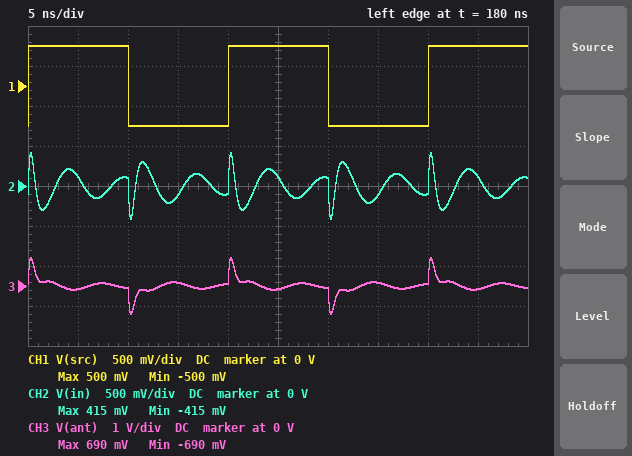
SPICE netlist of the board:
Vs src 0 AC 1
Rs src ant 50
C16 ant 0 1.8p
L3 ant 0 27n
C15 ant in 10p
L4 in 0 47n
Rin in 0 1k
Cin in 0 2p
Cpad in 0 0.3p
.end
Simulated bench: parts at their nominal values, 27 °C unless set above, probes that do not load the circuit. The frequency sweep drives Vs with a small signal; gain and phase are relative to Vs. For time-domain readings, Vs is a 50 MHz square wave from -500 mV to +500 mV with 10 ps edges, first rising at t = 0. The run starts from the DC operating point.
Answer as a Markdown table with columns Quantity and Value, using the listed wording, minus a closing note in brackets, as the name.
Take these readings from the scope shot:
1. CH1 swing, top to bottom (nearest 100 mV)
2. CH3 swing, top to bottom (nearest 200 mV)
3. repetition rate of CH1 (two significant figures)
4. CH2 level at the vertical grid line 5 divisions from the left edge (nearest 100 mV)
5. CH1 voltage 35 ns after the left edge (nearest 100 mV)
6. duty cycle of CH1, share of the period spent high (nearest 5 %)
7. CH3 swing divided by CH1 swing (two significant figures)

| Quantity | Value |
|---|---|
| CH1 swing, top to bottom | 1.0 V |
| CH3 swing, top to bottom | 1.4 V |
| repetition rate of CH1 | 50 MHz |
| CH2 level at the vertical grid line 5 divisions from the left edge | 100 mV |
| CH1 voltage 35 ns after the left edge | -500 mV |
| duty cycle of CH1, share of the period spent high | 50 % |
| CH3 swing divided by CH1 swing | 1.4 |
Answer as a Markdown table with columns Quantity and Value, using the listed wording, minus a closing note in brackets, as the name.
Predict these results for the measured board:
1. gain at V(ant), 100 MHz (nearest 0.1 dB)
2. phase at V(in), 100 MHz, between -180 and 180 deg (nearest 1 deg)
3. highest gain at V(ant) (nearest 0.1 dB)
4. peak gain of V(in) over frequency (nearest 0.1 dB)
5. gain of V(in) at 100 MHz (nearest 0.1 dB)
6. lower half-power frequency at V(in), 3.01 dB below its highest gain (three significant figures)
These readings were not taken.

| Quantity | Value |
|---|---|
| gain at V(ant), 100 MHz | -8.6 dB |
| phase at V(in), 100 MHz, between -180 and 180 deg | -114 deg |
| highest gain at V(ant) | -0.4 dB |
| peak gain of V(in) over frequency | 5.2 dB |
| gain of V(in) at 100 MHz | -21.0 dB |
| lower half-power frequency at V(in), 3.01 dB below its highest gain | 169 MHz |
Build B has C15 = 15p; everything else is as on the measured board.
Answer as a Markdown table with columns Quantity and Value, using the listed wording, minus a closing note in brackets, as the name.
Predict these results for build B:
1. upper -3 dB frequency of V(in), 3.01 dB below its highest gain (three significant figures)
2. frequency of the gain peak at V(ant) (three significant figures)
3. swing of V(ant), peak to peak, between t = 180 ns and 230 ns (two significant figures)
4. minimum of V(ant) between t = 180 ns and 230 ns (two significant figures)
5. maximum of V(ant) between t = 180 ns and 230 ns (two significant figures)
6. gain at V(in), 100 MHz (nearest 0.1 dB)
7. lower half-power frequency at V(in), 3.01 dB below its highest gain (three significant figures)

| Quantity | Value |
|---|---|
| upper -3 dB frequency of V(in), 3.01 dB below its highest gain | 172 MHz |
| frequency of the gain peak at V(ant) | 608 MHz |
| swing of V(ant), peak to peak, between t = 180 ns and 230 ns | 1.1 V |
| minimum of V(ant) between t = 180 ns and 230 ns | -570 mV |
| maximum of V(ant) between t = 180 ns and 230 ns | 570 mV |
| gain at V(in), 100 MHz | -15.5 dB |
| lower half-power frequency at V(in), 3.01 dB below its highest gain | 140 MHz |
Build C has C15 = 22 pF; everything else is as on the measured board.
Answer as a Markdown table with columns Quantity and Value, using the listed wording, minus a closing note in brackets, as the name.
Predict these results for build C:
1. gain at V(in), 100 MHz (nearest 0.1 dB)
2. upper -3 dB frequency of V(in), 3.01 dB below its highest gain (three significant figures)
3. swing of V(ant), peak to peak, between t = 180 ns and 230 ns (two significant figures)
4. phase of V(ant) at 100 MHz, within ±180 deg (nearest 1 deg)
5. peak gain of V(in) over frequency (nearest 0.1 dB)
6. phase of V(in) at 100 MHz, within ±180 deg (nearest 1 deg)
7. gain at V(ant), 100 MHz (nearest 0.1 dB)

| Quantity | Value |
|---|---|
| gain at V(in), 100 MHz | -8.5 dB |
| upper -3 dB frequency of V(in), 3.01 dB below its highest gain | 139 MHz |
| swing of V(ant), peak to peak, between t = 180 ns and 230 ns | 1.2 V |
| phase of V(ant) at 100 MHz, within ±180 deg | 59 deg |
| peak gain of V(in) over frequency | 4.4 dB |
| phase of V(in) at 100 MHz, within ±180 deg | -124 deg |
| gain at V(ant), 100 MHz | -5.9 dB |
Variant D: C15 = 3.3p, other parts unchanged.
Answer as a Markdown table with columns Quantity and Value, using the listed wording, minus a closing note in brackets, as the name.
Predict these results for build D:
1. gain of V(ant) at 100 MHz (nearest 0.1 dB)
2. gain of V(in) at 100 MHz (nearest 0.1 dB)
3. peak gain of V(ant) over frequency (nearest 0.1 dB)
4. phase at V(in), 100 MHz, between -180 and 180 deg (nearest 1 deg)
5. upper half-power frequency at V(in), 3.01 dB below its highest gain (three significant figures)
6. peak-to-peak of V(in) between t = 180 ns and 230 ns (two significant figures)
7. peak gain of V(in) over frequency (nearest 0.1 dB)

| Quantity | Value |
|---|---|
| gain of V(ant) at 100 MHz | -9.4 dB |
| gain of V(in) at 100 MHz | -32.7 dB |
| peak gain of V(ant) over frequency | -0.3 dB |
| phase at V(in), 100 MHz, between -180 and 180 deg | -112 deg |
| upper half-power frequency at V(in), 3.01 dB below its highest gain | 343 MHz |
| peak-to-peak of V(in) between t = 180 ns and 230 ns | 650 mV |
| peak gain of V(in) over frequency | 6.8 dB |
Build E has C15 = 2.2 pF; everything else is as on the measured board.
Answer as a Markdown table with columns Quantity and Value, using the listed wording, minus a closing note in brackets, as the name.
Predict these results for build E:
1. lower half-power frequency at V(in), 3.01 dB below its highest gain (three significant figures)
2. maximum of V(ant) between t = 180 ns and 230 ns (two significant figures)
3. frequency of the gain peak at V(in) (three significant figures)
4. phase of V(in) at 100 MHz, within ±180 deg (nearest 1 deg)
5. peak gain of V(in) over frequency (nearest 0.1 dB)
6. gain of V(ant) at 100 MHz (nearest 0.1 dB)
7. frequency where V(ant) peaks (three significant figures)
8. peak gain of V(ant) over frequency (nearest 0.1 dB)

| Quantity | Value |
|---|---|
| lower half-power frequency at V(in), 3.01 dB below its highest gain | 312 MHz |
| maximum of V(ant) between t = 180 ns and 230 ns | 700 mV |
| frequency of the gain peak at V(in) | 339 MHz |
| phase of V(in) at 100 MHz, within ±180 deg | -111 deg |
| peak gain of V(in) over frequency | 7.0 dB |
| gain of V(ant) at 100 MHz | -9.5 dB |
| frequency where V(ant) peaks | 637 MHz |
| peak gain of V(ant) over frequency | -0.2 dB |
